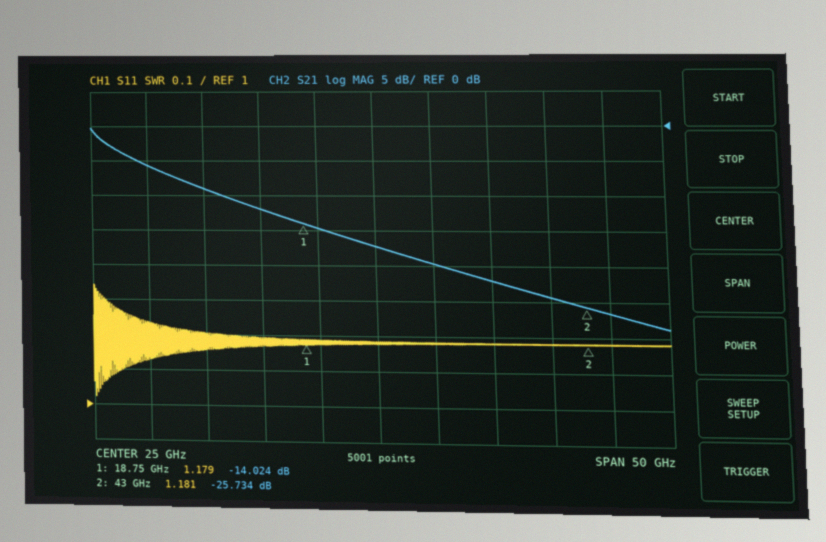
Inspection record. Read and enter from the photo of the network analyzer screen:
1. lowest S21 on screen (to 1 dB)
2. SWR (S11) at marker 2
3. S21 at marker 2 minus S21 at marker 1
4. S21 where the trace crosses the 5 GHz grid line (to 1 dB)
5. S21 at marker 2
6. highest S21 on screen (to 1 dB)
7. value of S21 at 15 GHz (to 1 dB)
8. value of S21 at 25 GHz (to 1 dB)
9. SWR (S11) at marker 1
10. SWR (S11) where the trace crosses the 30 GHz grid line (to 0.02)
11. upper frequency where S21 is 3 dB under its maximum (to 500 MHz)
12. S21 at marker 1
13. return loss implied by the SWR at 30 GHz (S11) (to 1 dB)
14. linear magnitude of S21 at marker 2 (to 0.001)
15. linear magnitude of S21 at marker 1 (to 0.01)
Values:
-29 dB
1.181
-11.710 dB
-6 dB
-25.734 dB
0 dB
-12 dB
-17 dB
1.179
1.18
2.0 GHz
-14.024 dB
22 dB
0.052
0.20
